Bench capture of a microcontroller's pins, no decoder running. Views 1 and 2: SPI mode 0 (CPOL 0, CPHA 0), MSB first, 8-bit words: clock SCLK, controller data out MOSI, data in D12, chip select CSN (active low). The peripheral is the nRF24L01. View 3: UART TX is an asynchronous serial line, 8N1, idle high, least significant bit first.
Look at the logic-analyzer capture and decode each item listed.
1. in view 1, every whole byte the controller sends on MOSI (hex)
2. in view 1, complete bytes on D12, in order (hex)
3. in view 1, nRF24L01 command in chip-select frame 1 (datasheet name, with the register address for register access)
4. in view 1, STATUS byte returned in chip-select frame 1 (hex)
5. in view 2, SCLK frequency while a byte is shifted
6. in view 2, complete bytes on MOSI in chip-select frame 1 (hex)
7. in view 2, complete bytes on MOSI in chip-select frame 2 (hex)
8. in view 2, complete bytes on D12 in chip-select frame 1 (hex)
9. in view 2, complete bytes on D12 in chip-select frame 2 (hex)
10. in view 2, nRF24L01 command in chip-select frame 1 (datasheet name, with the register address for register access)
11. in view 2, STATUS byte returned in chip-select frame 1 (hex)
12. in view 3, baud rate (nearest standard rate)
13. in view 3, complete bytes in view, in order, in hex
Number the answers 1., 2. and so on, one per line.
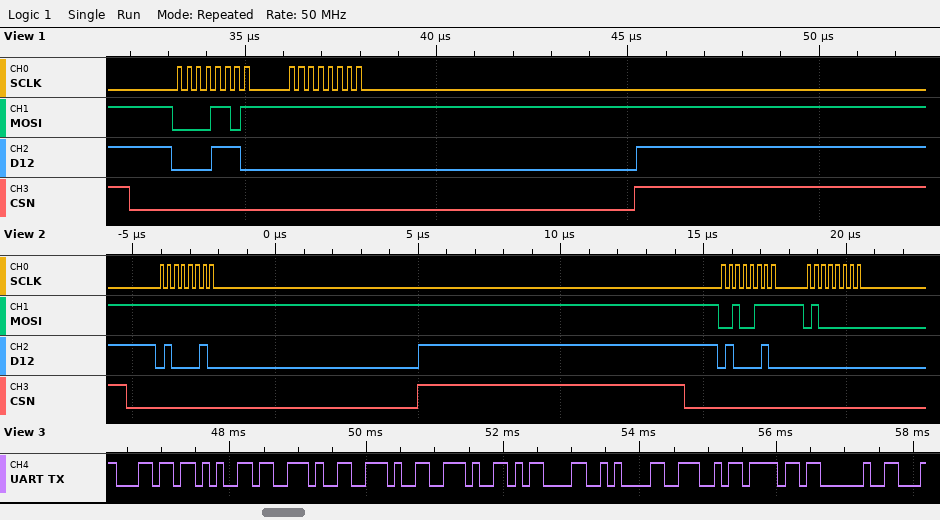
1. 0D FF
2. 0E 00
3. R_REGISTER 0x0D
4. 0x0E
5. 4 MHz
6. FF
7. 27 40
8. 42
9. 42 00
10. NOP
11. 0x42
12. 9600 baud
13. 0x6C 0x65 0x2E 0x2E 0x2E 0x0D 0x0A 0x4E 0x6F 0x20
